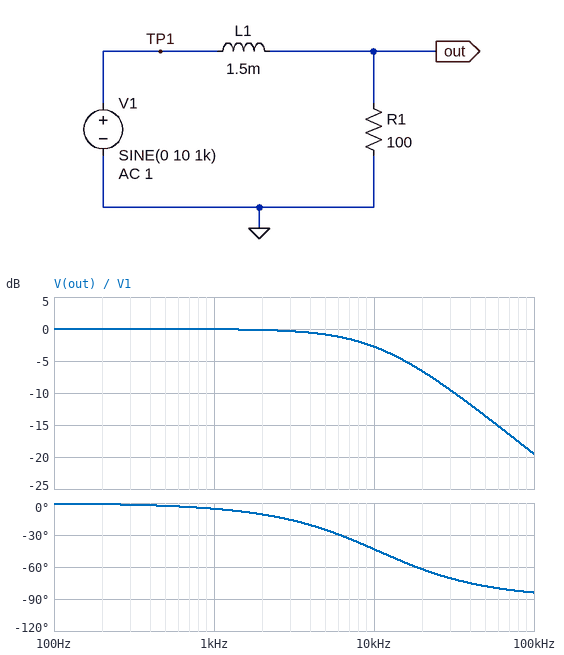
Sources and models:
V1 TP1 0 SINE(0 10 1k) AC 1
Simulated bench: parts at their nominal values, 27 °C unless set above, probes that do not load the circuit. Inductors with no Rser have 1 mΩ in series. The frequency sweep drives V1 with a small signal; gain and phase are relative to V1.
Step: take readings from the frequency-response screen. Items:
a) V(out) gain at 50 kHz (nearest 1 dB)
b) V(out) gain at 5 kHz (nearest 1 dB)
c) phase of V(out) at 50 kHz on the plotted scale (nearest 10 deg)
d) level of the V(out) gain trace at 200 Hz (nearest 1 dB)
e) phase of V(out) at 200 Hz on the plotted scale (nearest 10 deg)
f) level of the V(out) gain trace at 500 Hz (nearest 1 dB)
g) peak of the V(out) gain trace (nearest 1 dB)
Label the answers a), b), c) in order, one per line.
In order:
a) -14 dB
b) -1 dB
c) -80 deg
d) 0 dB
e) 0 deg
f) 0 dB
g) 0 dB
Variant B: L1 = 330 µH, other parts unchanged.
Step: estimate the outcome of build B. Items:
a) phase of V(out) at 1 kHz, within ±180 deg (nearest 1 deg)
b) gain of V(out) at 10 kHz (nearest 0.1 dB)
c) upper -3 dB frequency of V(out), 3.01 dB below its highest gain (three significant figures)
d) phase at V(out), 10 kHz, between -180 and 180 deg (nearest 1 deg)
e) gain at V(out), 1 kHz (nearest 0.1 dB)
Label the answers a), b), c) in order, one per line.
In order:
a) -1 deg
b) -0.2 dB
c) 48.2 kHz
d) -12 deg
e) 0 dB
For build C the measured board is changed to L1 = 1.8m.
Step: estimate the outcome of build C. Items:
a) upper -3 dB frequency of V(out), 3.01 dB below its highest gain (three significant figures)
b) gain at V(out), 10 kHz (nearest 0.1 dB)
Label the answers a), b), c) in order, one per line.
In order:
a) 8.84 kHz
b) -3.6 dB
